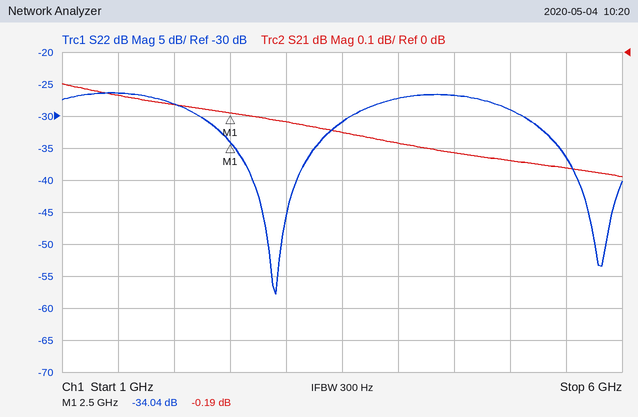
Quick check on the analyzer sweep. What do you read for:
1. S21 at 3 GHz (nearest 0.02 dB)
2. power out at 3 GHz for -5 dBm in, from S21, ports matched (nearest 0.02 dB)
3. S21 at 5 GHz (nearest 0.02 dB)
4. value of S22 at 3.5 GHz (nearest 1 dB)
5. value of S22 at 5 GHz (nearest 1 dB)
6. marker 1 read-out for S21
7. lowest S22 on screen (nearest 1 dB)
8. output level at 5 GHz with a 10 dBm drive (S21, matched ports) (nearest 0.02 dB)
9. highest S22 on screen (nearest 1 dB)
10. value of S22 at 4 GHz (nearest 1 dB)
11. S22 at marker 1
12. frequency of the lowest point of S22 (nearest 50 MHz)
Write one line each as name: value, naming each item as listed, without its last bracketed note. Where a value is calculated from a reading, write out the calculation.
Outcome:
S21 at 3 GHz: -0.22 dB
power out at 3 GHz for -5 dBm in, from S21, ports matched: -5 dBm + (-0.22 dB) = -5.22 dBm
S21 at 5 GHz: -0.34 dB
value of S22 at 3.5 GHz: -31 dB
value of S22 at 5 GHz: -29 dB
marker 1 read-out for S21: -0.19 dB
lowest S22 on screen: -58 dB
output level at 5 GHz with a 10 dBm drive (S21, matched ports): 10 dBm + (-0.34 dB) = 9.66 dBm
highest S22 on screen: -26 dB
value of S22 at 4 GHz: -27 dB
S22 at marker 1: -34.04 dB
frequency of the lowest point of S22: 2.90 GHz
